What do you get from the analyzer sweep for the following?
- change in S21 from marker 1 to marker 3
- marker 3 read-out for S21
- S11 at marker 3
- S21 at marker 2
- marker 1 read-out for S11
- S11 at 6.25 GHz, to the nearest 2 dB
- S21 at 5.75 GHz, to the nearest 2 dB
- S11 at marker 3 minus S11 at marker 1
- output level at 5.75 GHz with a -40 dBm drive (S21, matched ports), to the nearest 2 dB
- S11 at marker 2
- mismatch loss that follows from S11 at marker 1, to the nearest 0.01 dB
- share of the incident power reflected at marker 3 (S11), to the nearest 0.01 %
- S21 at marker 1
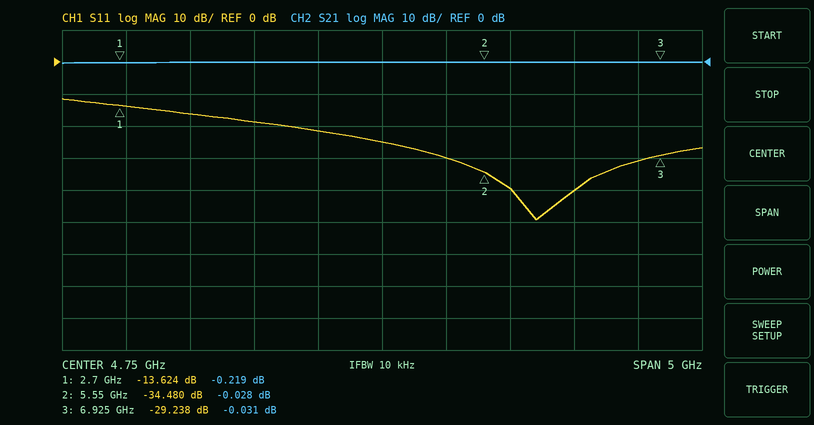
0.188 dB
-0.031 dB
-29.238 dB
-0.028 dB
-13.624 dB
-40 dB
0 dB
-15.614 dB
-40 dBm
-34.480 dB
0.19 dB
0.12 %
-0.219 dB
